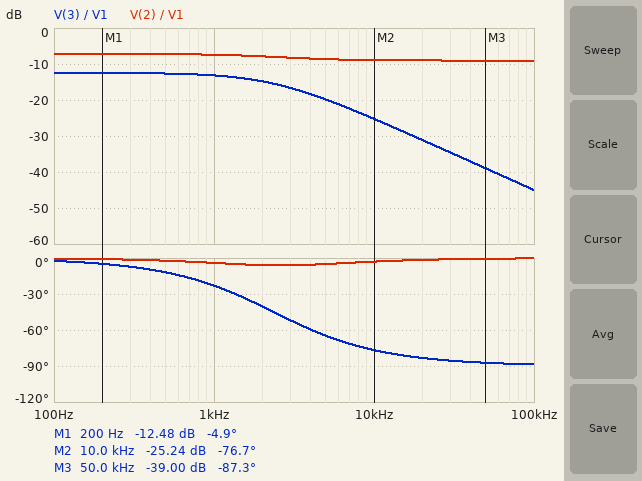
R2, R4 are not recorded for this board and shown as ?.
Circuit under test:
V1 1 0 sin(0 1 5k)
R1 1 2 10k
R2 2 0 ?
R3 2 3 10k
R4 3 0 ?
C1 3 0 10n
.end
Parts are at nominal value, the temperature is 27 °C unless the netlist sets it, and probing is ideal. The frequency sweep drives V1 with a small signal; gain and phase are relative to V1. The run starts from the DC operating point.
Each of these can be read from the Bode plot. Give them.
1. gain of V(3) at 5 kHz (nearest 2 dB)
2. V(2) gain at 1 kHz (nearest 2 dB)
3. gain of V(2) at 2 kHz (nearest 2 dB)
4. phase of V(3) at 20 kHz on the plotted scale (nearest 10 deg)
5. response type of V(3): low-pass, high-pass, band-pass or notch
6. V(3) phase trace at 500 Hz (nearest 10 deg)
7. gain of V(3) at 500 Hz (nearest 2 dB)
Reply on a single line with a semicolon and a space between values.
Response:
-20 dB; -8 dB; -8 dB; -80 deg; low-pass; -10 deg; -12 dB
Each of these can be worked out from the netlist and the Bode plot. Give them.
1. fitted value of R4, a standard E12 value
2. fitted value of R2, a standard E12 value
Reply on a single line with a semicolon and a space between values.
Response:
12 kΩ; 12 kΩ
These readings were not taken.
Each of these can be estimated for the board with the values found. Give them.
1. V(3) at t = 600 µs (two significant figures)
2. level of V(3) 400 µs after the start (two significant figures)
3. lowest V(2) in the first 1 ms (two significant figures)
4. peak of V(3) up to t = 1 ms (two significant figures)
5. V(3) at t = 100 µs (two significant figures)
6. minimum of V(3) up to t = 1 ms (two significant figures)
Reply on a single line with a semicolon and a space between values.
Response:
-92 mV; -92 mV; -370 mV; 130 mV; 110 mV; -100 mV
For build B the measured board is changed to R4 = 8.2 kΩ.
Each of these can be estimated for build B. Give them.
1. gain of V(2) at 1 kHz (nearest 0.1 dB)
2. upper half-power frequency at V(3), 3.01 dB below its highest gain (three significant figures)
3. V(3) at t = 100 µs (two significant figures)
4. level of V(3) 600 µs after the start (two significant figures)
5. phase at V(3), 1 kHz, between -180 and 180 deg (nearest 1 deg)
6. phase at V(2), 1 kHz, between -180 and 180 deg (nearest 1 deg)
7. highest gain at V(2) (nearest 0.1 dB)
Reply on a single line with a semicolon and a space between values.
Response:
-7.7 dB; 2.97 kHz; 96 mV; -83 mV; -19 deg; -3 deg; -7.5 dB
